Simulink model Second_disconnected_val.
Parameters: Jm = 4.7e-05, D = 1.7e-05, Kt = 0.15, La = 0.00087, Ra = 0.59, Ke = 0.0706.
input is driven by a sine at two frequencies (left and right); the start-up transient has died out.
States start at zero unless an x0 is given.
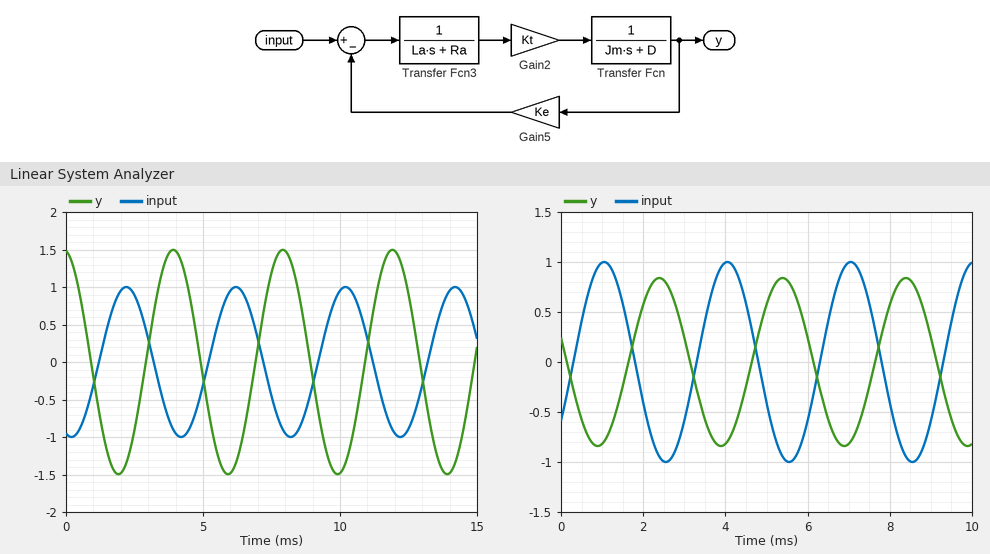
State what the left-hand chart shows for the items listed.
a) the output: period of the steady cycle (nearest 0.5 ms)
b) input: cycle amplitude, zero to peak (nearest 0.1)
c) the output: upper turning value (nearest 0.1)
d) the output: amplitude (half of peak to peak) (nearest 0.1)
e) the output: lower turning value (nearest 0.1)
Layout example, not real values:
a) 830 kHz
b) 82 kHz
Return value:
a) 4.0 ms
b) 1.0
c) 1.5
d) 1.5
e) -1.5
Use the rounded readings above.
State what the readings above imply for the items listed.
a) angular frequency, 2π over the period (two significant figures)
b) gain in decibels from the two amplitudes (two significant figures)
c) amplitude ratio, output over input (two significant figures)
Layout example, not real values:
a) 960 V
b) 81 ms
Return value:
a) 1.6 rad/ms
b) 3.5 dB
c) 1.5
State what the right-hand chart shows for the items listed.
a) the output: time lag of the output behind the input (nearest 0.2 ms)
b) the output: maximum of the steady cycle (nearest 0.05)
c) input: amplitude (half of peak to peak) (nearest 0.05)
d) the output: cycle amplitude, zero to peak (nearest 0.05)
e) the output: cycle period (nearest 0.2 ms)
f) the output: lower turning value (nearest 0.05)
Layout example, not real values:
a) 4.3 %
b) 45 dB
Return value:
a) 1.4 ms
b) 0.85
c) 1.00
d) 0.85
e) 3.0 ms
f) -0.85
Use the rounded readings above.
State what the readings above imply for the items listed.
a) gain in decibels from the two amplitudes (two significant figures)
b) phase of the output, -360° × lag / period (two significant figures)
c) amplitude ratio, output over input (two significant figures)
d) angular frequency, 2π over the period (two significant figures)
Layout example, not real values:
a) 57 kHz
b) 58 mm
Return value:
a) -1.4 dB
b) -170°
c) 0.85
d) 2.1 rad/ms
